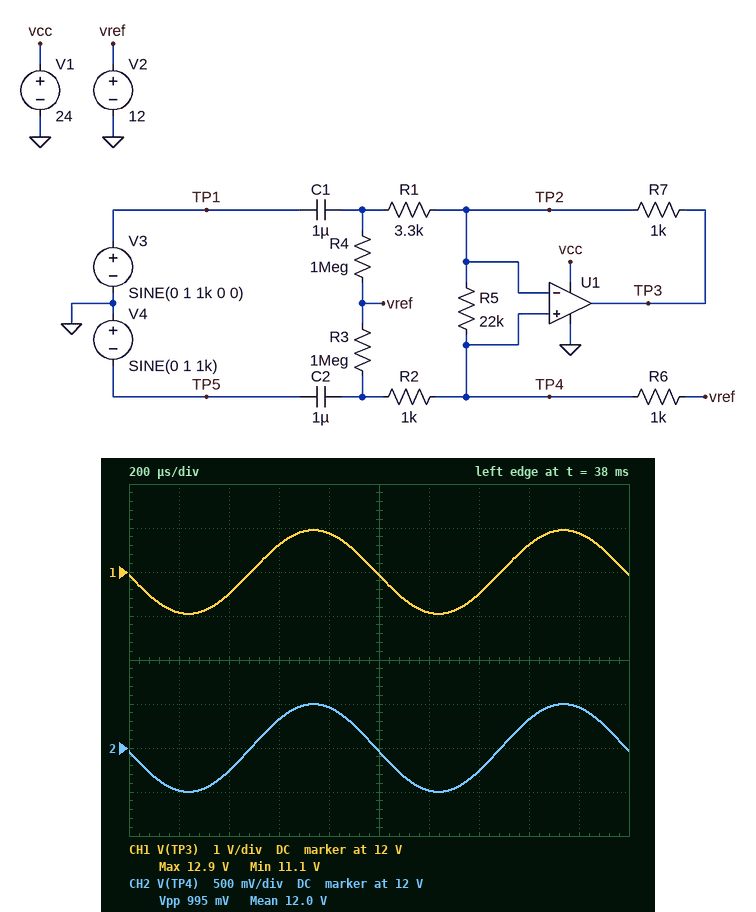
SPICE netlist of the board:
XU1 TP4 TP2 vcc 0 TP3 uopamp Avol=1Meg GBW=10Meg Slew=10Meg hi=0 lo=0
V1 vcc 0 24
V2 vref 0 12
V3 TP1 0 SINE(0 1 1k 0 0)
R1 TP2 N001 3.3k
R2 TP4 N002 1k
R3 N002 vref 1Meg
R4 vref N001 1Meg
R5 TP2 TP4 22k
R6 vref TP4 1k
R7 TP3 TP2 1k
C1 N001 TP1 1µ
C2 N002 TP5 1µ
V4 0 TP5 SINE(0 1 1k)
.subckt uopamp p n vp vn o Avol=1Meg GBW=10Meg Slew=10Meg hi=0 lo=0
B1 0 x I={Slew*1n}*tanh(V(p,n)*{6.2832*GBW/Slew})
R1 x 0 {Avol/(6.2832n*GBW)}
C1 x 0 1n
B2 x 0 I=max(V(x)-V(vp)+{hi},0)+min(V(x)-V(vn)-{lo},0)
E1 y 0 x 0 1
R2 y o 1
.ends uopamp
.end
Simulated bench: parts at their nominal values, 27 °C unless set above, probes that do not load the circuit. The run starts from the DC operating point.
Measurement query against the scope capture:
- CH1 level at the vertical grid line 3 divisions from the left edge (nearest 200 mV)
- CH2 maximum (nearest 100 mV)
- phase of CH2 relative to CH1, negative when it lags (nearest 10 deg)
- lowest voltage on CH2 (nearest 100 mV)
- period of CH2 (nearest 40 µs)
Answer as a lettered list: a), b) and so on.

a) 12.6 V
b) 12.5 V
c) 0 deg
d) 11.5 V
e) 1.00 ms
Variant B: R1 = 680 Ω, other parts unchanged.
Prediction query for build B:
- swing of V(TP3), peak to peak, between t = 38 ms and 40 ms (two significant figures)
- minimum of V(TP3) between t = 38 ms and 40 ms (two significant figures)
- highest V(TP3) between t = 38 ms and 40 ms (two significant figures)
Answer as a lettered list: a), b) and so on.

a) 5.3 V
b) 9.4 V
c) 15 V
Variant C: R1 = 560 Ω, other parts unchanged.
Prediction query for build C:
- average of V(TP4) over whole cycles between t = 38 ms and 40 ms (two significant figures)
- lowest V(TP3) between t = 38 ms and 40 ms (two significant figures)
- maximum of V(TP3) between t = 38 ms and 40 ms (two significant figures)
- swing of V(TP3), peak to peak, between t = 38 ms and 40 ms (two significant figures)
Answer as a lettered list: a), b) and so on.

a) 12 V
b) 8.9 V
c) 15 V
d) 6.1 V
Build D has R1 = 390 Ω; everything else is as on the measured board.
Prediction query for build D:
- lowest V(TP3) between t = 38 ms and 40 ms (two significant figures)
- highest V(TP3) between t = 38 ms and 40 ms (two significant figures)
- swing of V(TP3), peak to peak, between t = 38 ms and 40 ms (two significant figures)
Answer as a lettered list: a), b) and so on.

a) 8.0 V
b) 16 V
c) 8.1 V
